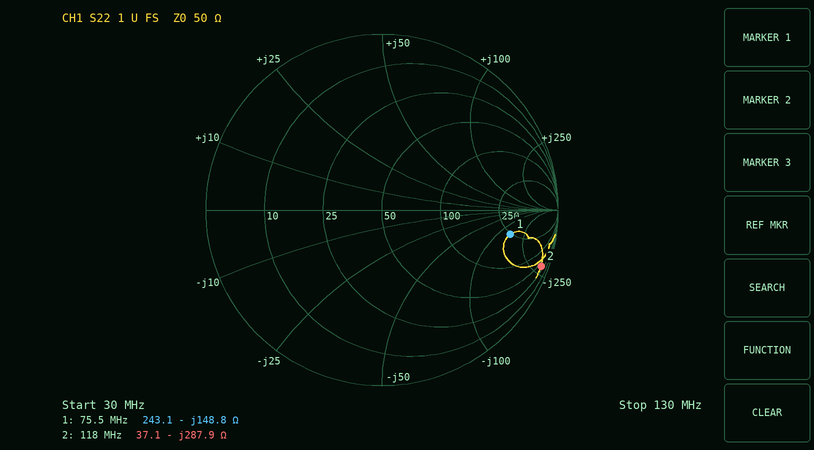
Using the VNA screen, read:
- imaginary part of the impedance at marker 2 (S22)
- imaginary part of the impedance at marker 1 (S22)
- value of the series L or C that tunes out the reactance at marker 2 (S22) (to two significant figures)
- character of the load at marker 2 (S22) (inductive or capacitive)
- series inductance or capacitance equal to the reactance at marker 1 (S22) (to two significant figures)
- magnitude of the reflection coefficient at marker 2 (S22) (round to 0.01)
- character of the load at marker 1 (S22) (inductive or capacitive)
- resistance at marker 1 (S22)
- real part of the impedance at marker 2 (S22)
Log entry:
-287.9 Ω
-148.8 Ω
390 nH
capacitive
14 pF
0.96
capacitive
243.1 Ω
37.1 Ω
